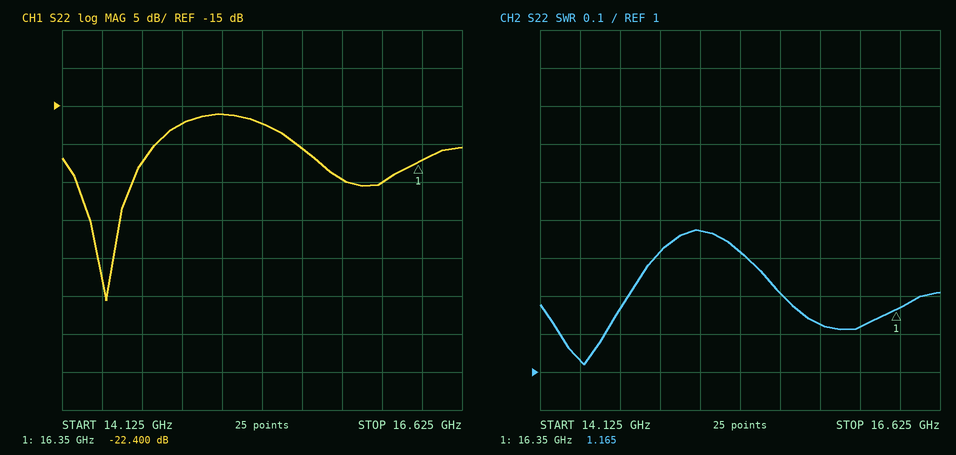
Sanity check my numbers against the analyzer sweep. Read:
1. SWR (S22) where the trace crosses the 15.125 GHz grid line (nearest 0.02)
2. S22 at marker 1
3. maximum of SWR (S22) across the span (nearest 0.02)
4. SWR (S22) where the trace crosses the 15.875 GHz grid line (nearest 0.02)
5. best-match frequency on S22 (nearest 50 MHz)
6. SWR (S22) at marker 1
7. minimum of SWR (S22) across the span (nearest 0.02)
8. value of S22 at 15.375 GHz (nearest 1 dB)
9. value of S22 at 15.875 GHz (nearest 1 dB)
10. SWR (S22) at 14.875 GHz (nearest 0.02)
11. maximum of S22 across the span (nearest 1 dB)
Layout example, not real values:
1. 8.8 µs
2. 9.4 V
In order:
1. 1.38
2. -22.400 dB
3. 1.38
4. 1.12
5. 14.40 GHz
6. 1.165
7. 1.02
8. -17 dB
9. -25 dB
10. 1.32
11. -16 dB
